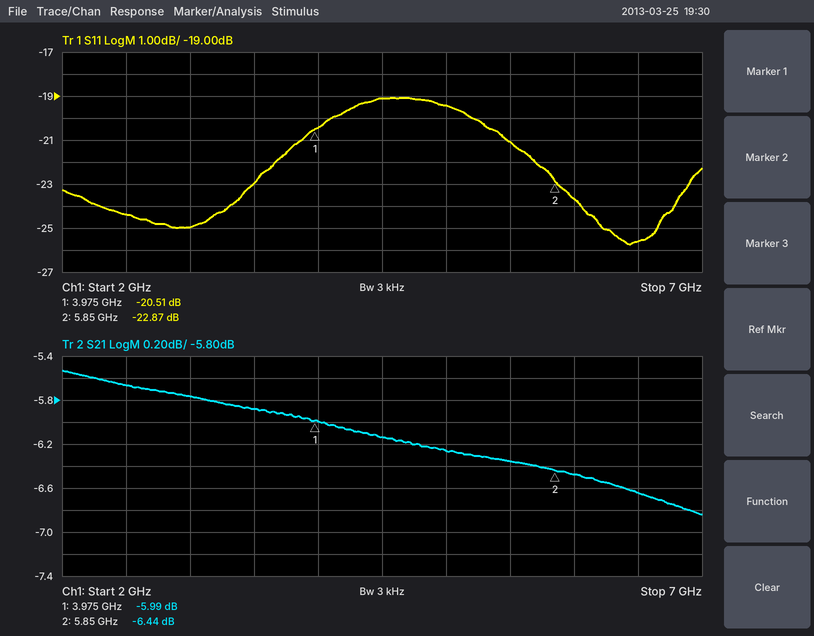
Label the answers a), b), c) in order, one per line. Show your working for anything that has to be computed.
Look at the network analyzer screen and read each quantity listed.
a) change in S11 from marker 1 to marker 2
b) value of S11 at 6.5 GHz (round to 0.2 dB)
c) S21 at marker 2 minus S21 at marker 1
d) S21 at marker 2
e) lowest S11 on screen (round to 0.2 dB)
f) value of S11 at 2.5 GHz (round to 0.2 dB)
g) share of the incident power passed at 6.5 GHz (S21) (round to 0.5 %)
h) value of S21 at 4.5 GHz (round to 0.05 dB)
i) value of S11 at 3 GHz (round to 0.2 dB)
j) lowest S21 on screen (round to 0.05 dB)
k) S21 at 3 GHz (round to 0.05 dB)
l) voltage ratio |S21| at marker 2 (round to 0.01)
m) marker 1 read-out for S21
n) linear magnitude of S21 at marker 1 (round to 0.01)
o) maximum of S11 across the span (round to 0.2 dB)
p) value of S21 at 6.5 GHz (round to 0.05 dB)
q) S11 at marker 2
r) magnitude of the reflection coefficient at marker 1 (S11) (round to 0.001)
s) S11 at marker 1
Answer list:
a) -22.87 − (-20.51) = -2.36 dB
b) -25.6 dB
c) -6.44 − (-5.99) = -0.45 dB
d) -6.44 dB
e) -25.8 dB
f) -24.4 dB
g) 10^(-6.65/10) ≈ 21.6 %, so 21.5 % to the nearest 0.5 %
h) -6.15 dB
i) -25.0 dB
j) -6.85 dB
k) -5.75 dB
l) 10^(-6.44/20) ≈ 0.48
m) -5.99 dB
n) 10^(-5.99/20) ≈ 0.50
o) -19.0 dB
p) -6.65 dB
q) -22.87 dB
r) 10^(-20.51/20) ≈ 0.094
s) -20.51 dB
